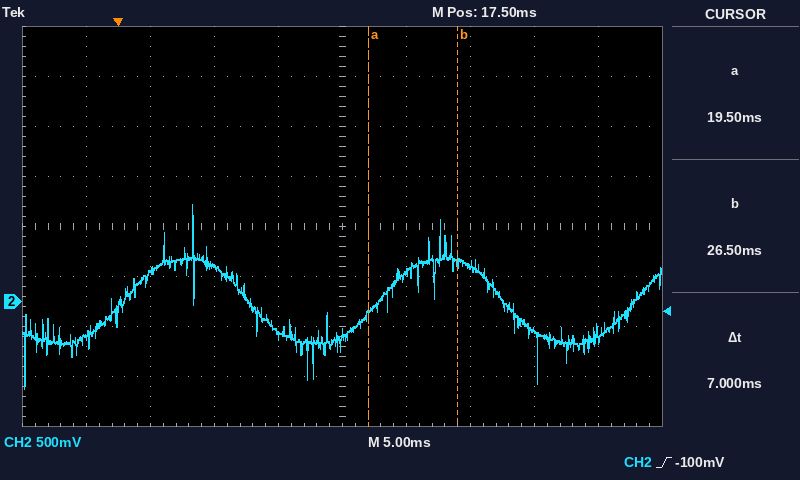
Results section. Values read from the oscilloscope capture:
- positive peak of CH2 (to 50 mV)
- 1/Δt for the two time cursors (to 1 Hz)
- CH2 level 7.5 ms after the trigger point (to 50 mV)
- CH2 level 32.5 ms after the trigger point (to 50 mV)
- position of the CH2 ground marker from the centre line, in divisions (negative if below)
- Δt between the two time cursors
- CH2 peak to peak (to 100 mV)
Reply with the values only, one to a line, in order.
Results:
950 mV
143 Hz
350 mV
-300 mV
-1.5 div
7 ms
1.80 V
